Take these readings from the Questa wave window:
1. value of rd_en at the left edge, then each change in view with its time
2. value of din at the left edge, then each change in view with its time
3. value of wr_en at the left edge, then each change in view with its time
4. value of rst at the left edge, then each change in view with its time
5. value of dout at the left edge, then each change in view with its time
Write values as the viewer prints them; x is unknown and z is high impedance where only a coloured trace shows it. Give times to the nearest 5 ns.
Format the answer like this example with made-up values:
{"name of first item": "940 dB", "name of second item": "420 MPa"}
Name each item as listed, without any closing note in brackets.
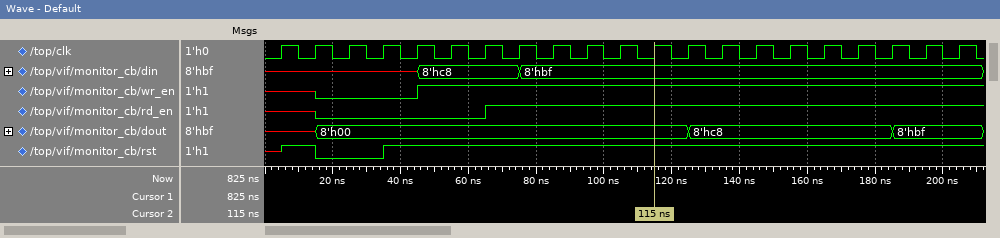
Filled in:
{"value of rd_en at the left edge, then each change in view with its time": "x, 0 at 15 ns, 1 at 65 ns", "value of din at the left edge, then each change in view with its time": "x, 8'hc8 at 45 ns, 8'hbf at 75 ns", "value of wr_en at the left edge, then each change in view with its time": "x, 0 at 15 ns, 1 at 45 ns", "value of rst at the left edge, then each change in view with its time": "x, 1 at 5 ns, 0 at 15 ns, 1 at 35 ns", "value of dout at the left edge, then each change in view with its time": "x, 8'h00 at 15 ns, 8'hc8 at 125 ns, 8'hbf at 185 ns"}
